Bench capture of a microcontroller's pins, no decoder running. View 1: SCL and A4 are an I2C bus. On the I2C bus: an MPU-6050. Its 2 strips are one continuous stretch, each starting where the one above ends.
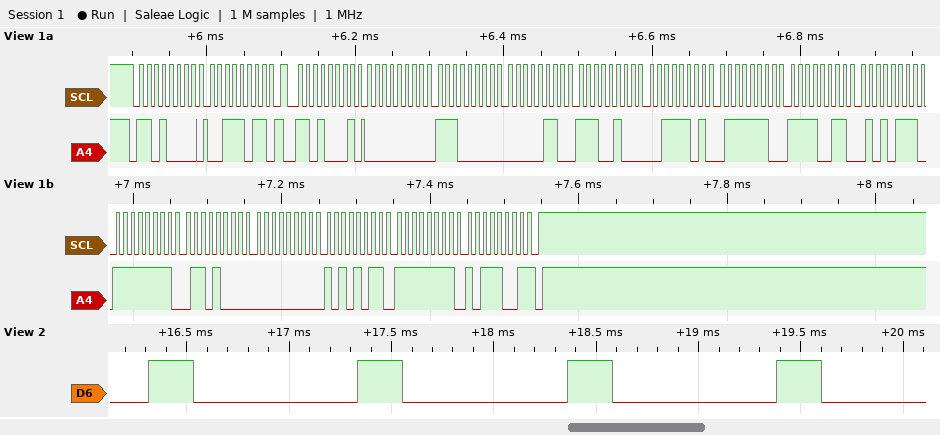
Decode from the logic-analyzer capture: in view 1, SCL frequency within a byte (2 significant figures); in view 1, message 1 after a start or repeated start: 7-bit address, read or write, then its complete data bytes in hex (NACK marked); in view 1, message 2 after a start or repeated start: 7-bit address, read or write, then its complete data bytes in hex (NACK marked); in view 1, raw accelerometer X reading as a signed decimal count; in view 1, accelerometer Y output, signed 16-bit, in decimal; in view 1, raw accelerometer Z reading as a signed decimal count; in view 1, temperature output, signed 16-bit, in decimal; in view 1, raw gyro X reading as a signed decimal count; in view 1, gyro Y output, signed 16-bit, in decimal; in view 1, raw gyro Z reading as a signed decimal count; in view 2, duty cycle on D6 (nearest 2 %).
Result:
100 kHz
0x68 write: 3B
0x68 read: 00 E0 06 E4 3D 7E F3 57 FF 68 00 AB FF B9 NACK
224
1764
15742
-3241
-152
171
-71
22 %
